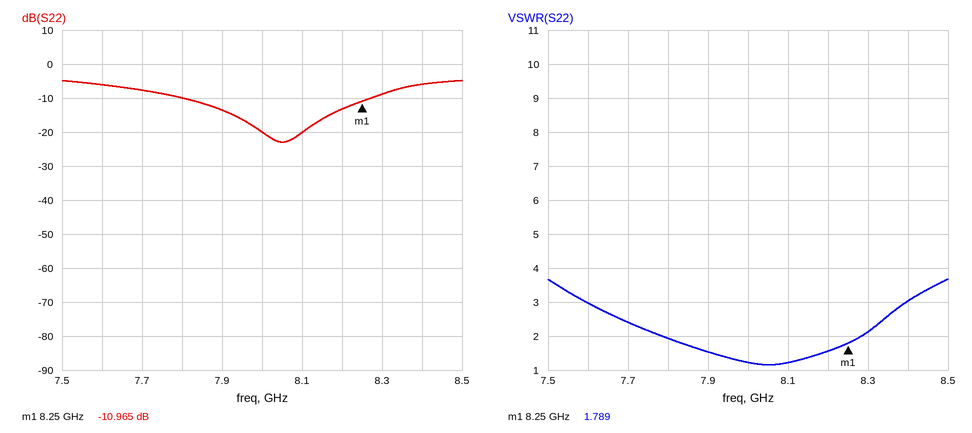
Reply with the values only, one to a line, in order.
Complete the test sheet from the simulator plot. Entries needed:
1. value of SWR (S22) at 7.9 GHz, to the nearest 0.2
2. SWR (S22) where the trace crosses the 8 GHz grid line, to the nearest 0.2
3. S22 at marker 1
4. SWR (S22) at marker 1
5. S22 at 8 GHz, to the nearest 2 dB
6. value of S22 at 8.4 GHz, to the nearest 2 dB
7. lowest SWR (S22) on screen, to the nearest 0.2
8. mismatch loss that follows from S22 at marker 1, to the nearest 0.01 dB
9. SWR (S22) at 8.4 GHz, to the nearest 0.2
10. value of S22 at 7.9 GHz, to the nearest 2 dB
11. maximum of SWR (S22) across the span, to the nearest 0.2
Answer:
1.6
1.2
-10.965 dB
1.789
-20 dB
-6 dB
1.2
0.36 dB
3.0
-14 dB
3.6
